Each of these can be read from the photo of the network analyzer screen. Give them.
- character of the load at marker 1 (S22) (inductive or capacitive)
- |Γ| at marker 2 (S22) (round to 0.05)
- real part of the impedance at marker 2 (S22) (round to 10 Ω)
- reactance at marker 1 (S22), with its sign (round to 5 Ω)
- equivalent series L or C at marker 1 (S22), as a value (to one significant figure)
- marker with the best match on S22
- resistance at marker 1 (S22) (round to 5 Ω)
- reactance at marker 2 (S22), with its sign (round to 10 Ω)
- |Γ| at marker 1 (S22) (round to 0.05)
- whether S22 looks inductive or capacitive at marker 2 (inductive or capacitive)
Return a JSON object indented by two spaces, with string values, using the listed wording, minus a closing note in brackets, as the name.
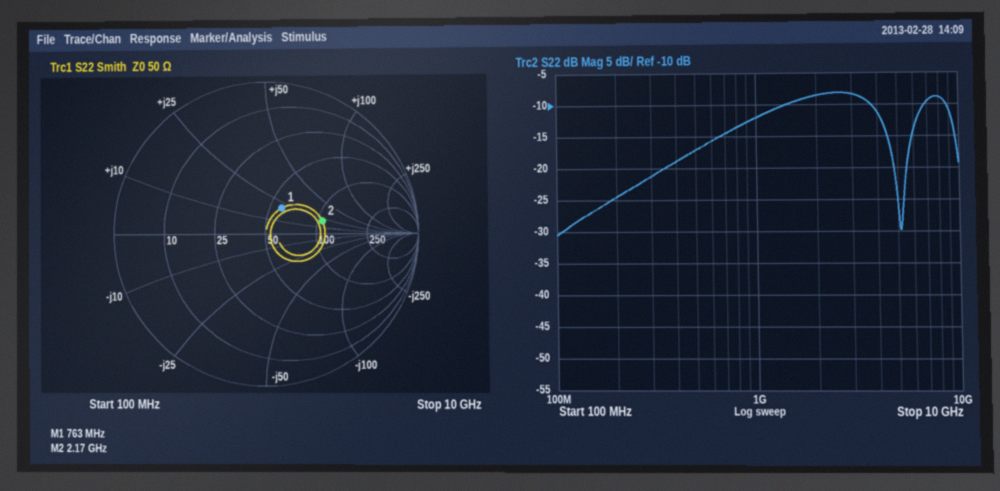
{
  "character of the load at marker 1 (S22)": "inductive",
  "|Γ| at marker 2 (S22)": "0.40",
  "real part of the impedance at marker 2 (S22)": "110 Ω",
  "reactance at marker 1 (S22), with its sign": "+20 Ω",
  "equivalent series L or C at marker 1 (S22), as a value": "4 nH",
  "marker with the best match on S22": "marker 1",
  "resistance at marker 1 (S22)": "60 Ω",
  "reactance at marker 2 (S22), with its sign": "+20 Ω",
  "|Γ| at marker 1 (S22)": "0.20",
  "whether S22 looks inductive or capacitive at marker 2": "inductive"
}
